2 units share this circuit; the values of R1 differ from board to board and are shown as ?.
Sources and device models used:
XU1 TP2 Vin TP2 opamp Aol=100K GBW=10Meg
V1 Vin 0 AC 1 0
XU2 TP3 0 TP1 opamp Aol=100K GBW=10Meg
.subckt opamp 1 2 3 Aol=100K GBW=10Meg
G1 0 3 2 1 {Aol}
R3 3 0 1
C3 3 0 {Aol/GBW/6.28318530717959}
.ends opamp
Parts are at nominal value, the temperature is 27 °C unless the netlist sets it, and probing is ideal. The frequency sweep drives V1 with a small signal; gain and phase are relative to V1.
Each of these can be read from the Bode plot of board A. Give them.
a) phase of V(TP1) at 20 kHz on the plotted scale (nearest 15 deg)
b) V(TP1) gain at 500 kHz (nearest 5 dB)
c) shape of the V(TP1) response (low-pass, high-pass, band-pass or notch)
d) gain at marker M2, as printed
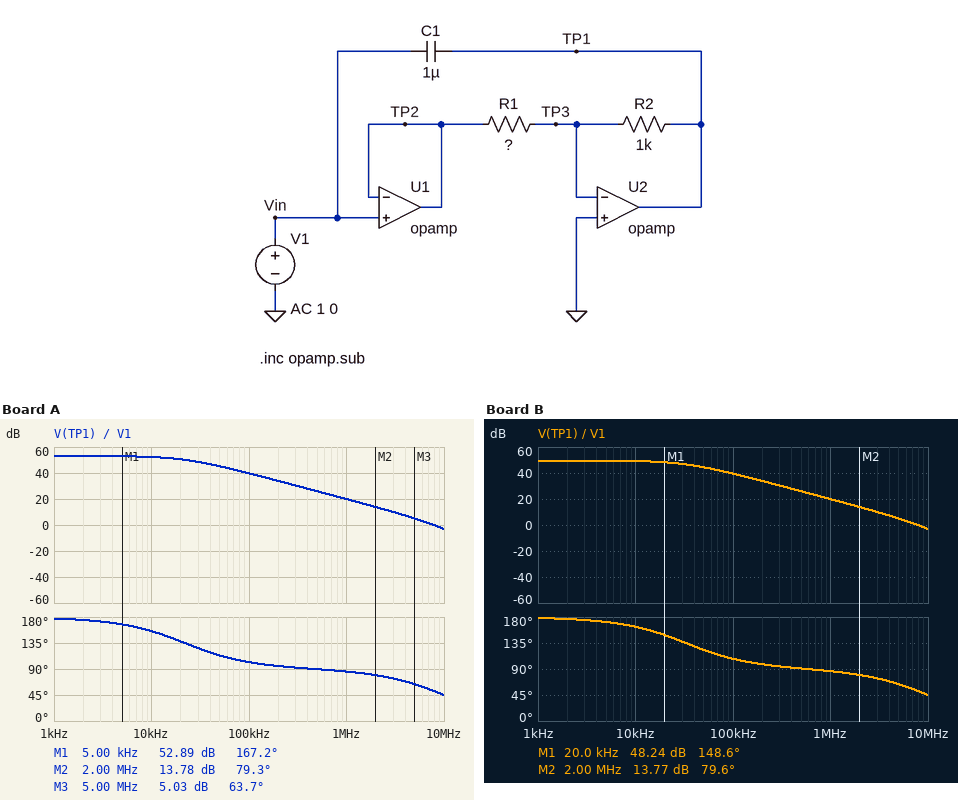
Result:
135 deg
25 dB
low-pass
13.78 dB
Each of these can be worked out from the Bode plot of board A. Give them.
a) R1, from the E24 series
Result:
2.2 Ω
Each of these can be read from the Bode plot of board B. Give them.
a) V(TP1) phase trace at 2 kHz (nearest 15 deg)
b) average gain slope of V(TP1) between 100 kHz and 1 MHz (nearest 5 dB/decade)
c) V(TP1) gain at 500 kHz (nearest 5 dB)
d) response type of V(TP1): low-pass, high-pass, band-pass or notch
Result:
180 deg
-20 dB/decade
25 dB
low-pass
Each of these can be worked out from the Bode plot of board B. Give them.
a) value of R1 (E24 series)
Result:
3.3 Ω
